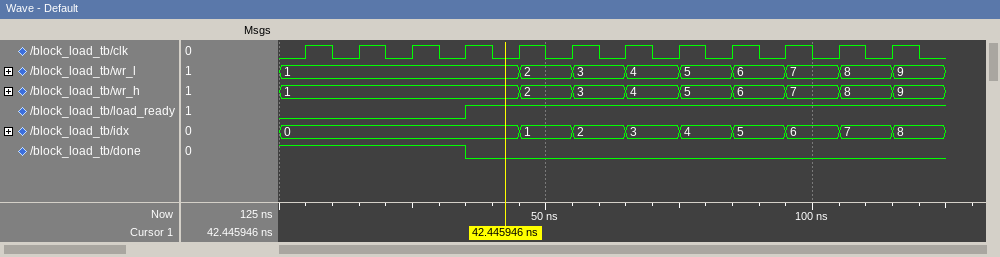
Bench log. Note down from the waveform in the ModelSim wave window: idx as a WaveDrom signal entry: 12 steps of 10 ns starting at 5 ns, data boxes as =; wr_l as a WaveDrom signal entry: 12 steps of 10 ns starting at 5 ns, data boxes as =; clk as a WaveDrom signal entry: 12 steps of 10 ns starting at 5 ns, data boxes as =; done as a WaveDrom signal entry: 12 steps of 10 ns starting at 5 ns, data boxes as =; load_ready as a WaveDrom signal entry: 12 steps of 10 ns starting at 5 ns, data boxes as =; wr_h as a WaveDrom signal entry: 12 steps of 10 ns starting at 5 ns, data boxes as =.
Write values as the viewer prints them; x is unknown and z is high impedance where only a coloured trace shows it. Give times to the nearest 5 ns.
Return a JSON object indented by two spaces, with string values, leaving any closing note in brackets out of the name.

{
  "idx as a WaveDrom signal entry: 12 steps of 10 ns starting at 5 ns, data boxes as =": "{name: 'idx', wave: '=...========', data: '0 1 2 3 4 5 6 7 8'}",
  "wr_l as a WaveDrom signal entry: 12 steps of 10 ns starting at 5 ns, data boxes as =": "{name: 'wr_l', wave: '=...========', data: '1 2 3 4 5 6 7 8 9'}",
  "clk as a WaveDrom signal entry: 12 steps of 10 ns starting at 5 ns, data boxes as =": "{name: 'clk', wave: 'p...........'}",
  "done as a WaveDrom signal entry: 12 steps of 10 ns starting at 5 ns, data boxes as =": "{name: 'done', wave: '1..0........'}",
  "load_ready as a WaveDrom signal entry: 12 steps of 10 ns starting at 5 ns, data boxes as =": "{name: 'load_ready', wave: '0..1........'}",
  "wr_h as a WaveDrom signal entry: 12 steps of 10 ns starting at 5 ns, data boxes as =": "{name: 'wr_h', wave: '=...========', data: '1 2 3 4 5 6 7 8 9'}"
}
